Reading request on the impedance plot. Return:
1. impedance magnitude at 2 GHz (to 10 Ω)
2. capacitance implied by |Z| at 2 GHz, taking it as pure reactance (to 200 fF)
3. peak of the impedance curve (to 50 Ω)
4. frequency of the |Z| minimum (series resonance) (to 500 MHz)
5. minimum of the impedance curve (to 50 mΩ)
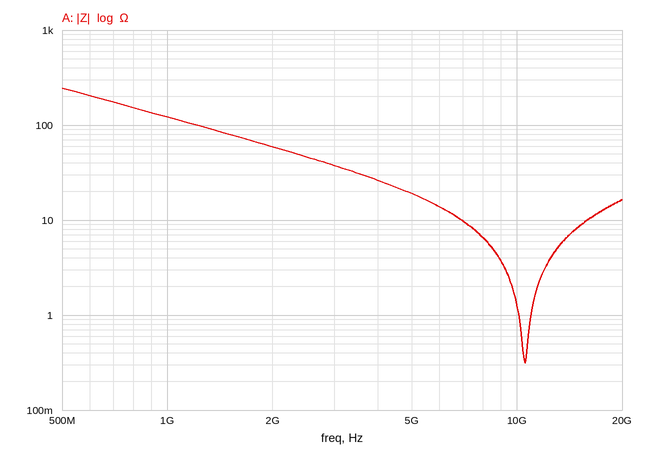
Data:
60 Ω
1.4 pF
250 Ω
10.5 GHz
300 mΩ
